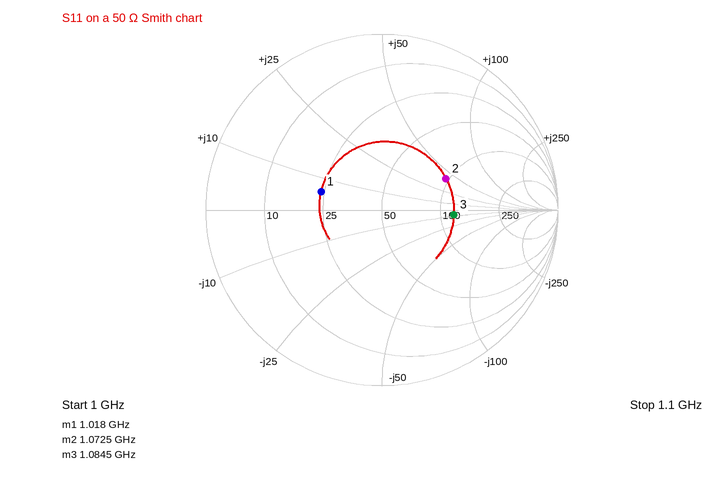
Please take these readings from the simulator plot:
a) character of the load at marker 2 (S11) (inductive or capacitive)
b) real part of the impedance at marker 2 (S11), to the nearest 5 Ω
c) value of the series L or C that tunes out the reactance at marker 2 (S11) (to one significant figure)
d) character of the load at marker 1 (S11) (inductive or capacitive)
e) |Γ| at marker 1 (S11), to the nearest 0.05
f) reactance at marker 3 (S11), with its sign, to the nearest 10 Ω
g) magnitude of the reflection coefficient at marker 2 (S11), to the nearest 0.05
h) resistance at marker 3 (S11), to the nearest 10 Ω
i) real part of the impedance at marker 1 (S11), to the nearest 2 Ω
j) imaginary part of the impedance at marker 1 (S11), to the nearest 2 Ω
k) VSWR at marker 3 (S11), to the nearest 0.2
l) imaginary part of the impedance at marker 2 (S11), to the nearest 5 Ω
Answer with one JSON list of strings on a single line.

["inductive", "95 Ω", "4 pF", "inductive", "0.35", "-10 Ω", "0.40", "120 Ω", "24 Ω", "+6 Ω", "2.4", "+40 Ω"]
